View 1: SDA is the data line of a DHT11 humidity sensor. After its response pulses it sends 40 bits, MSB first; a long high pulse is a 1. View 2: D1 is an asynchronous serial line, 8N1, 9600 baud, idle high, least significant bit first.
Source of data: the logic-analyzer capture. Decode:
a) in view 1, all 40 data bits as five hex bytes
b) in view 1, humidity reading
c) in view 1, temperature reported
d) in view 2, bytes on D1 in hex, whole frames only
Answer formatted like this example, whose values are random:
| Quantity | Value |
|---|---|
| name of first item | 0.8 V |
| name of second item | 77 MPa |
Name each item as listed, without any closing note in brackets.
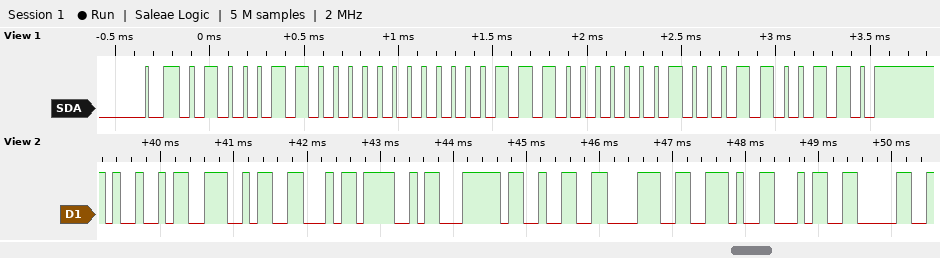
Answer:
| Quantity | Value |
|---|---|
| in view 1, all 40 data bits as five hex bytes | 46 00 1C 04 66 |
| in view 1, humidity reading | 70 % |
| in view 1, temperature reported | 28.4 °C |
| in view 2, bytes on D1 in hex, whole frames only | 49 4E 46 4F 7C 32 38 2E 34 30 |
